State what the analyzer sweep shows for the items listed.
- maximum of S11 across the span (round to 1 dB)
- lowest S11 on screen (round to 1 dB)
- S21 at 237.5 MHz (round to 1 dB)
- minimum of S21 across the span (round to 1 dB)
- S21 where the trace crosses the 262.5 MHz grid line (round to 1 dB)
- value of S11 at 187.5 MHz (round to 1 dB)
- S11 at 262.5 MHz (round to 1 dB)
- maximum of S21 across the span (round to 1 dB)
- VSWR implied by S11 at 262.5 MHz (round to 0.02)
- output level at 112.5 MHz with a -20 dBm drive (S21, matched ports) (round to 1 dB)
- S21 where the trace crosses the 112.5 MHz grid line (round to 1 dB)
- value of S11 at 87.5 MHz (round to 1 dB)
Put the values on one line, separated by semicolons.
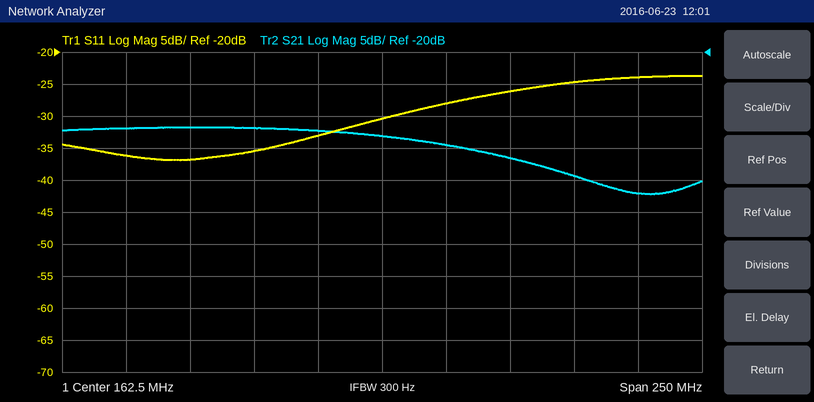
-24 dB; -37 dB; -39 dB; -42 dB; -42 dB; -28 dB; -24 dB; -32 dB; 1.14; -52 dBm; -32 dB; -37 dB
